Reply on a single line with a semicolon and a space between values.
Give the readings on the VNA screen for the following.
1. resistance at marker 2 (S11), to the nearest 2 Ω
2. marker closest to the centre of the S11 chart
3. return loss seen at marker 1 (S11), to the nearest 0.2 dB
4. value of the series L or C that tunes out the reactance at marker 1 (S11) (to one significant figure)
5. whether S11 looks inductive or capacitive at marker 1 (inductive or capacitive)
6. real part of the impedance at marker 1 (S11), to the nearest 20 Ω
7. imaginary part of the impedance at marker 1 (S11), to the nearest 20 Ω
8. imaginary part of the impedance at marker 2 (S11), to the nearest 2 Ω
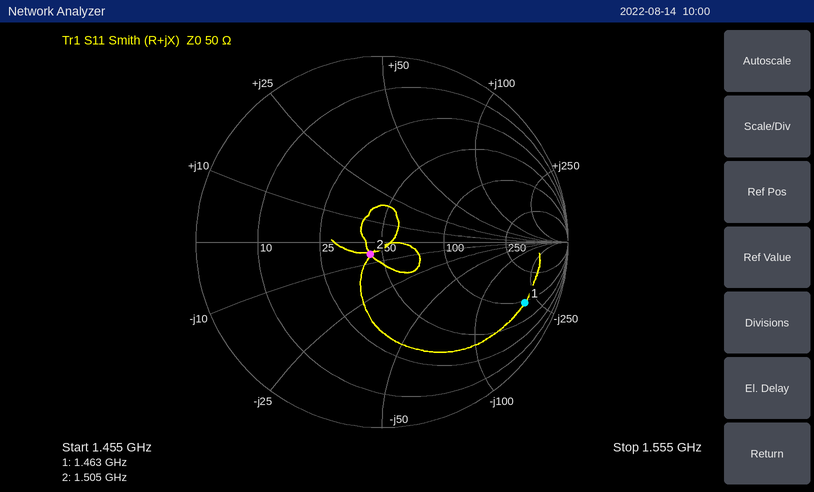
44 Ω; marker 2; 1.6 dB; 20 nH; capacitive; 100 Ω; -200 Ω; -6 Ω
